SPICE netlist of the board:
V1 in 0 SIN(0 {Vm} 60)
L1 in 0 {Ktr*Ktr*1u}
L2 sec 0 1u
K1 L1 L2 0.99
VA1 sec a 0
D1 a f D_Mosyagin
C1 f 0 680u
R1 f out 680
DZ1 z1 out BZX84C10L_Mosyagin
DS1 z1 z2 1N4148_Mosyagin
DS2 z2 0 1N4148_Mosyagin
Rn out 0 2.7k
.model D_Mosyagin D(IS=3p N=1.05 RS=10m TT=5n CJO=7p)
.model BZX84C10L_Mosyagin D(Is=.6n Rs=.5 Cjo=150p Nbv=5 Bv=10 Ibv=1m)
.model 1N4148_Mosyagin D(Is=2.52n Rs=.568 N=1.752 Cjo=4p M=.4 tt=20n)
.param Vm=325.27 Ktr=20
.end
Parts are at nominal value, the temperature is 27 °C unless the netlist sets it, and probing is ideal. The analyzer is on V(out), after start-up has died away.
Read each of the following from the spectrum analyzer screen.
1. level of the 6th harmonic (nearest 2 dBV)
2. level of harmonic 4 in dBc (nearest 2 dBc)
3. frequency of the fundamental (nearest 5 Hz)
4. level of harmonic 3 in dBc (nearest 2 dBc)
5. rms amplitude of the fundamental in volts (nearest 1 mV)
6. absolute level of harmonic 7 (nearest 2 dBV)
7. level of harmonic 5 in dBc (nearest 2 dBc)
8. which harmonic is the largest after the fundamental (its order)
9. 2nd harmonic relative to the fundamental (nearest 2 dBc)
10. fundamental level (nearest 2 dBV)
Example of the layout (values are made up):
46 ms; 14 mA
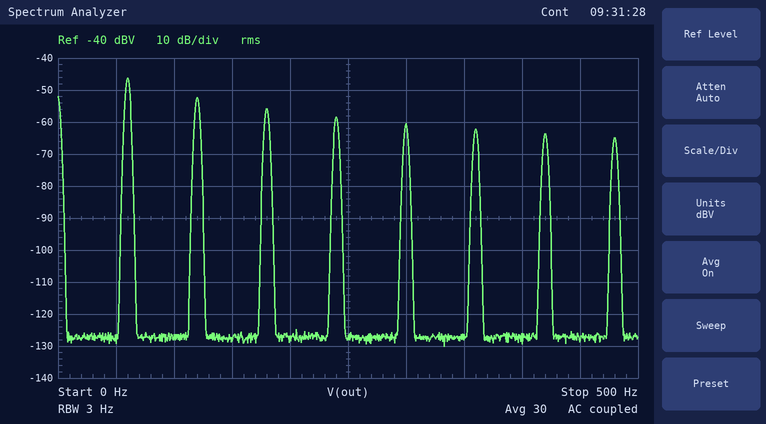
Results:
-62 dBV; -12 dBc; 60 Hz; -10 dBc; 5 mV; -64 dBV; -14 dBc; 2; -6 dBc; -46 dBV
